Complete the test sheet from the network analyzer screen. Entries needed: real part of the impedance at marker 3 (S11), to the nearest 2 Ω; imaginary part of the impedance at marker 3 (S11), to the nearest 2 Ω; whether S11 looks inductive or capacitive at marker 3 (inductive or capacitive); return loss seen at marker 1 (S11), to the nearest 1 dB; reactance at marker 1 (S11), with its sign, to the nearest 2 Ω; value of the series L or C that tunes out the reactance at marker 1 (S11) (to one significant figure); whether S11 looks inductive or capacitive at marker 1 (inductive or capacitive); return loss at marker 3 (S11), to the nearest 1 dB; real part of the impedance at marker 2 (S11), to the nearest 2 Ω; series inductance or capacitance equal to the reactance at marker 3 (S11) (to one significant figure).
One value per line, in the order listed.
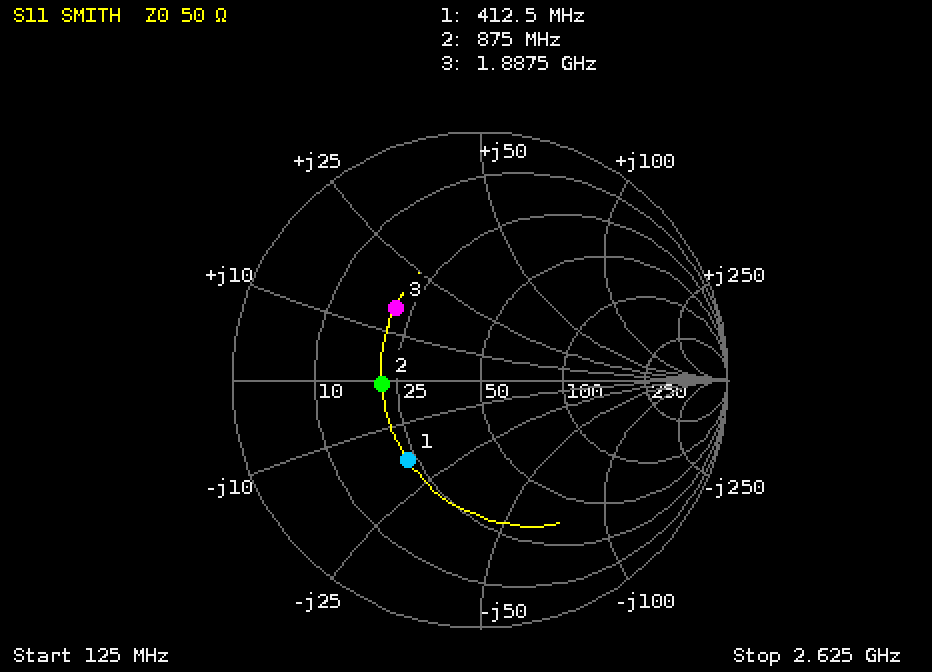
22 Ω
+16 Ω
inductive
7 dB
-18 Ω
7 nH
capacitive
7 dB
22 Ω
1 nH
